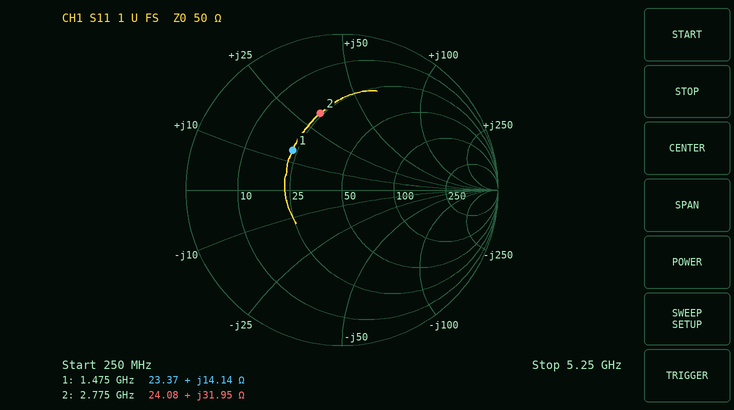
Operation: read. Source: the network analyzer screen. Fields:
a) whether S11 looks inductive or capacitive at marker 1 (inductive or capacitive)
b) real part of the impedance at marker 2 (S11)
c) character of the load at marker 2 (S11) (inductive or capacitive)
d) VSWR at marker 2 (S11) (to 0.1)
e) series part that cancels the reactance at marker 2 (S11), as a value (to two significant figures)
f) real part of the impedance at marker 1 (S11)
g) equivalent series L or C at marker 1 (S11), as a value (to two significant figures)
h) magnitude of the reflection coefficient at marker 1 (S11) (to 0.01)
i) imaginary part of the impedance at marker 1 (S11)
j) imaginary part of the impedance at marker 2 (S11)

inductive
24.08 Ω
inductive
3.1
1.8 pF
23.37 Ω
1.5 nH
0.40
+14.14 Ω
+31.95 Ω
